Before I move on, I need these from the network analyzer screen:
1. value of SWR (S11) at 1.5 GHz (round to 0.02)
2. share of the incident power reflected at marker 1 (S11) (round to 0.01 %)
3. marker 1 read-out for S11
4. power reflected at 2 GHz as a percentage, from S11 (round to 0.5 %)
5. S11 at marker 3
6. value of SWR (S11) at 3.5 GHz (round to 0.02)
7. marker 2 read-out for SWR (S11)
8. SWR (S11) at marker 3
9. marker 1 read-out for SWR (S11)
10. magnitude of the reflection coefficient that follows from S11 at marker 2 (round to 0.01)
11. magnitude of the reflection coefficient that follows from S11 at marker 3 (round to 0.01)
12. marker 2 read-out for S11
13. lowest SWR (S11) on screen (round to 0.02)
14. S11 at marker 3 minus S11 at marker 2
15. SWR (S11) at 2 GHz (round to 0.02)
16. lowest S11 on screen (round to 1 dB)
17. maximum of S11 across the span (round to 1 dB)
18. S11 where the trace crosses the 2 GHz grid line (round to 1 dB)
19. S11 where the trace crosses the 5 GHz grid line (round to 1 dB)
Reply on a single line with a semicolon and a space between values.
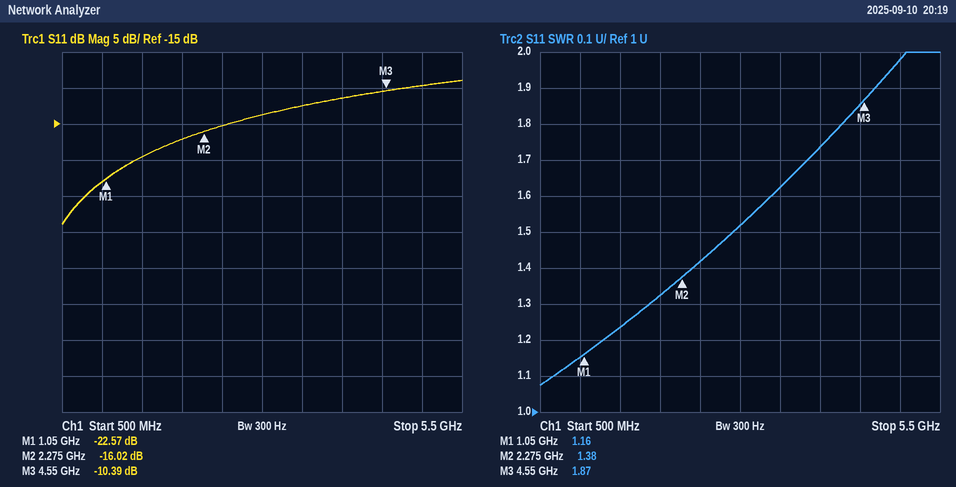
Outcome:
1.24; 0.55 %; -22.57 dB; 2.0 %; -10.39 dB; 1.62; 1.38; 1.87; 1.16; 0.16; 0.30; -16.02 dB; 1.08; 5.63 dB; 1.32; -29 dB; -9 dB; -17 dB; -10 dB
